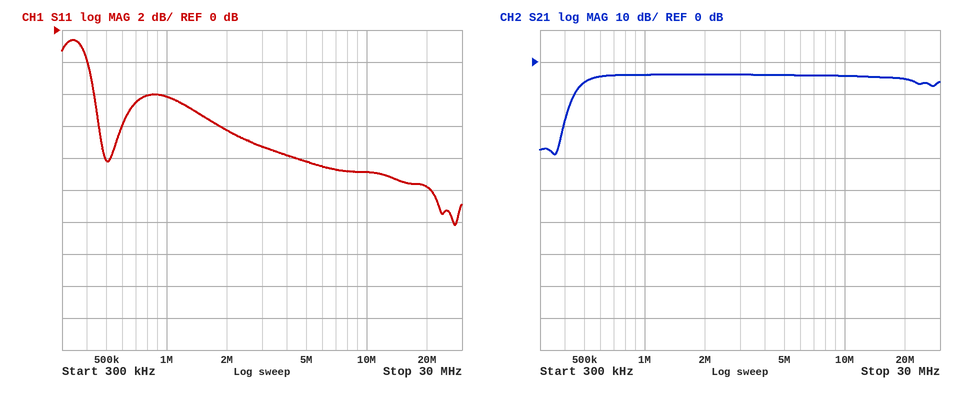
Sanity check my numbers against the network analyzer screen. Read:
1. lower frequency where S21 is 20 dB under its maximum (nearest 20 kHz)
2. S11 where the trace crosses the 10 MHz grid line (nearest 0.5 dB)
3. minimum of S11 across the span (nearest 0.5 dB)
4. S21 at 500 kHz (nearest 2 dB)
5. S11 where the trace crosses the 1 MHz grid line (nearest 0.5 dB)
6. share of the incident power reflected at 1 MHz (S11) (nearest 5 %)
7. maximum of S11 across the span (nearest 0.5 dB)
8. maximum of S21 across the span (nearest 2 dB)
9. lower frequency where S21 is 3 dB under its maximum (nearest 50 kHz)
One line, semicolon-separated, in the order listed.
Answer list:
380 kHz; -9.0 dB; -12.0 dB; -6 dB; -4.0 dB; 40 %; -0.5 dB; -4 dB; 500 kHz
